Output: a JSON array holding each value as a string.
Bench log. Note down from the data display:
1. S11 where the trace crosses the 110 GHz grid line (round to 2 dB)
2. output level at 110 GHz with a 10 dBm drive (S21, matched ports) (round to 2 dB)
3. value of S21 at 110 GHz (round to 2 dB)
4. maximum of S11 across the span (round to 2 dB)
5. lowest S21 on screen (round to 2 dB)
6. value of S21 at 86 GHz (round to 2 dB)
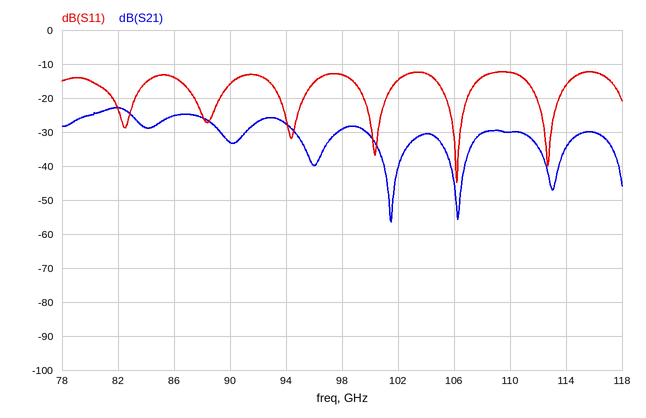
["-12 dB", "-20 dBm", "-30 dB", "-12 dB", "-56 dB", "-26 dB"]
